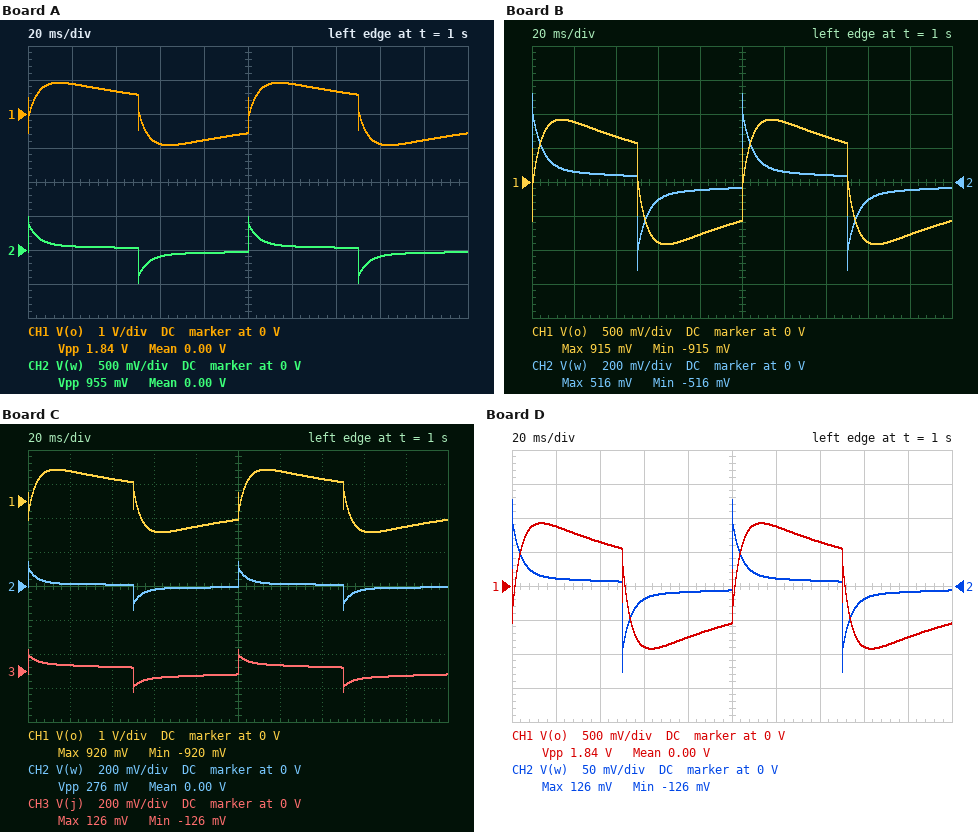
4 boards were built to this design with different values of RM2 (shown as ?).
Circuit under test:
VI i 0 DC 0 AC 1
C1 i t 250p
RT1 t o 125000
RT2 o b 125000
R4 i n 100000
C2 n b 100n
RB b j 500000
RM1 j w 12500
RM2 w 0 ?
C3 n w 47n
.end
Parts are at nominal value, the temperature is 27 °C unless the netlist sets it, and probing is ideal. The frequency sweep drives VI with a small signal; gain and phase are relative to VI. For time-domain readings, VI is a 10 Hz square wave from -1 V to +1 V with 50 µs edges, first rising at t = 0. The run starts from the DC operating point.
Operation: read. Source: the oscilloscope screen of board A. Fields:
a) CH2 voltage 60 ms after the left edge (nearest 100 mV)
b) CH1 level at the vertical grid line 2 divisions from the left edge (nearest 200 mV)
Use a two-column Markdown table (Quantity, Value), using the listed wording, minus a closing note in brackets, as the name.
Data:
| Quantity | Value |
|---|---|
| CH2 voltage 60 ms after the left edge | -100 mV |
| CH1 level at the vertical grid line 2 divisions from the left edge | 600 mV |
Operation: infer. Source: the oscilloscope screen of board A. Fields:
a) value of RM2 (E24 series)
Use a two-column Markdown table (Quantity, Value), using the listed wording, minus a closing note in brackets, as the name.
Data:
| Quantity | Value |
|---|---|
| value of RM2 | 27 kΩ |
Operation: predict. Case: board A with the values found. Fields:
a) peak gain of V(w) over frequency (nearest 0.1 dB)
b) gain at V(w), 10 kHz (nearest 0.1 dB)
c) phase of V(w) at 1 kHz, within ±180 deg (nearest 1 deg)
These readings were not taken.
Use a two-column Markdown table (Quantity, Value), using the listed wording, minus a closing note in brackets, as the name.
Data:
| Quantity | Value |
|---|---|
| peak gain of V(w) over frequency | -11.2 dB |
| gain at V(w), 10 kHz | -11.3 dB |
| phase of V(w) at 1 kHz, within ±180 deg | 7 deg |
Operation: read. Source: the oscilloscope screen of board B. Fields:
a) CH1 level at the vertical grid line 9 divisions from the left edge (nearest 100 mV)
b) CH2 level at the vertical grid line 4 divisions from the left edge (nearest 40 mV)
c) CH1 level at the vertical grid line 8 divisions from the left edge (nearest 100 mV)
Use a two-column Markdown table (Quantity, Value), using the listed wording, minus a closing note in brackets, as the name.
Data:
| Quantity | Value |
|---|---|
| CH1 level at the vertical grid line 9 divisions from the left edge | -800 mV |
| CH2 level at the vertical grid line 4 divisions from the left edge | -40 mV |
| CH1 level at the vertical grid line 8 divisions from the left edge | -900 mV |
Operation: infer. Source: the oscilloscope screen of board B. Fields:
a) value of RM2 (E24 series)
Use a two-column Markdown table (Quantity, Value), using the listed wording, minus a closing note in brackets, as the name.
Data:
| Quantity | Value |
|---|---|
| value of RM2 | 30 kΩ |
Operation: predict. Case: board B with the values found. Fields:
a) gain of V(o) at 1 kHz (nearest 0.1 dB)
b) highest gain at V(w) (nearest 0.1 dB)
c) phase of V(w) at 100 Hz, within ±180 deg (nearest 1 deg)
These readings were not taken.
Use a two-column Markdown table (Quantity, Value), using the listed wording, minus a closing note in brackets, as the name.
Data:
| Quantity | Value |
|---|---|
| gain of V(o) at 1 kHz | -9.8 dB |
| highest gain at V(w) | -10.6 dB |
| phase of V(w) at 100 Hz, within ±180 deg | 15 deg |
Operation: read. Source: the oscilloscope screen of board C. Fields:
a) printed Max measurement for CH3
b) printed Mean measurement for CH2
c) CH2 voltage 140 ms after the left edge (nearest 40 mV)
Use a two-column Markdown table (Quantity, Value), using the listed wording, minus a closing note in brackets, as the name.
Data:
| Quantity | Value |
|---|---|
| printed Max measurement for CH3 | 126 mV |
| printed Mean measurement for CH2 | 0.00 V |
| CH2 voltage 140 ms after the left edge | 0 V |
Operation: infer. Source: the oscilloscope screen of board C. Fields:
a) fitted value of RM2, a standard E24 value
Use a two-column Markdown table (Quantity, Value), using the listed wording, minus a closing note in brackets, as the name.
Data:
| Quantity | Value |
|---|---|
| fitted value of RM2, a standard E24 value | 6.2 kΩ |
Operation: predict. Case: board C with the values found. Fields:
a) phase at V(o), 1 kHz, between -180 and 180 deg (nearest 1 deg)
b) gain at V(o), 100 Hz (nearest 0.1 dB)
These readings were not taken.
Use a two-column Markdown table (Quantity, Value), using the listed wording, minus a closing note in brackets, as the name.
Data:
| Quantity | Value |
|---|---|
| phase at V(o), 1 kHz, between -180 and 180 deg | 47 deg |
| gain at V(o), 100 Hz | -10.7 dB |
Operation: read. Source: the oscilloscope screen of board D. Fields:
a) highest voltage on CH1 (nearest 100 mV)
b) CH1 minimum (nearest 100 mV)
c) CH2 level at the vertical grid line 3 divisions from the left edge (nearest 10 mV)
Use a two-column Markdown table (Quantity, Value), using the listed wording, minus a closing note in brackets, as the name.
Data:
| Quantity | Value |
|---|---|
| highest voltage on CH1 | 900 mV |
| CH1 minimum | -900 mV |
| CH2 level at the vertical grid line 3 divisions from the left edge | -20 mV |
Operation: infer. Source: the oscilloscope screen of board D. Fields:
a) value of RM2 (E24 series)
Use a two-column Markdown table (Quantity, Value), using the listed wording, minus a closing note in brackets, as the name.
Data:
| Quantity | Value |
|---|---|
| value of RM2 | 5.6 kΩ |
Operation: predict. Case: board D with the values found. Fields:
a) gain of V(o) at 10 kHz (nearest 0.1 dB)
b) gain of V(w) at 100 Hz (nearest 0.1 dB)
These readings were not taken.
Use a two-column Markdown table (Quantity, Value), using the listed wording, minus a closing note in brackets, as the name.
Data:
| Quantity | Value |
|---|---|
| gain of V(o) at 10 kHz | -5.7 dB |
| gain of V(w) at 100 Hz | -26.1 dB |
